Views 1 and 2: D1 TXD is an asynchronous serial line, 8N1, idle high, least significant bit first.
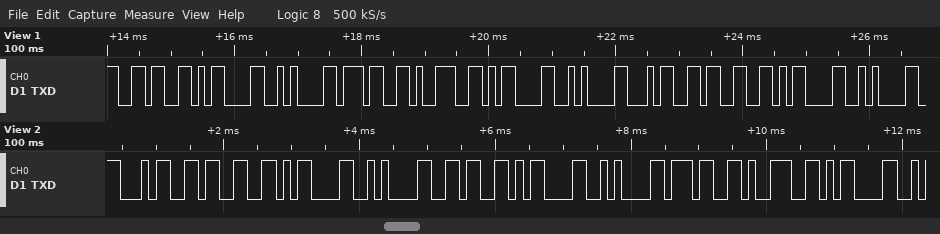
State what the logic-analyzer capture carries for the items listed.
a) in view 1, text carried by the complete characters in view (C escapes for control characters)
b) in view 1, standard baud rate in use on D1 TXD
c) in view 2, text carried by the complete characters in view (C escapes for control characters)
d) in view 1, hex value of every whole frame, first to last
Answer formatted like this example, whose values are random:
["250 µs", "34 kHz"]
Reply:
["\"6\\r\\n79\\r\\n43\\r\\n\"", "9600 baud", "\"43\\r\\n6\\r\\n79\\r\"", "0x36 0x0D 0x0A 0x37 0x39 0x0D 0x0A 0x34 0x33 0x0D 0x0A"]
